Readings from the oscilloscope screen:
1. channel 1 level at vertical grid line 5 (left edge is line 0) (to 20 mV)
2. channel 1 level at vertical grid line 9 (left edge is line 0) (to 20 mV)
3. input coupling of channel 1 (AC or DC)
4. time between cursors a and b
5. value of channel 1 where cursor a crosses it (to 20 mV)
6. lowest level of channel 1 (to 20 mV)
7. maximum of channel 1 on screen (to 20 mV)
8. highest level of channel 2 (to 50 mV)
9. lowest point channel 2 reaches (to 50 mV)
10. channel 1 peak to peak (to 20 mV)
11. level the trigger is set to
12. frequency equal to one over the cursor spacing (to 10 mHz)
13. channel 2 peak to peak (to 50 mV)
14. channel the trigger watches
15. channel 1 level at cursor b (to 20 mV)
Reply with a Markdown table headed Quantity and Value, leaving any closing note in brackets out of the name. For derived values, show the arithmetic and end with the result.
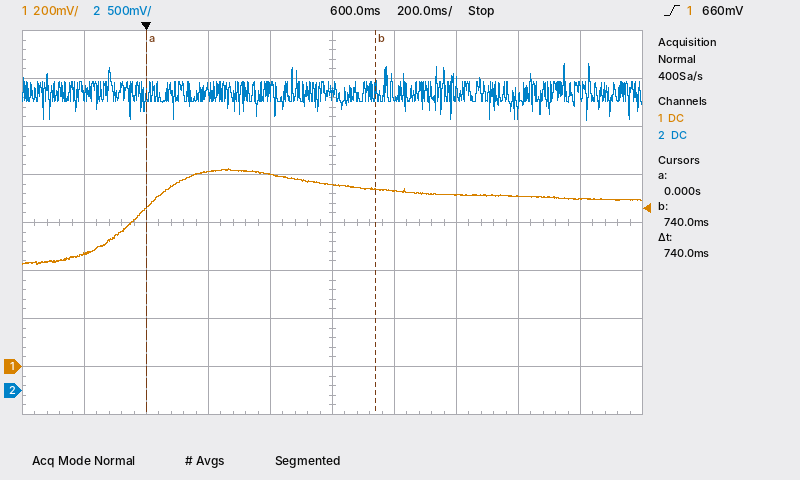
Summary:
| Quantity | Value |
|---|---|
| channel 1 level at vertical grid line 5 (left edge is line 0) | 760 mV |
| channel 1 level at vertical grid line 9 (left edge is line 0) | 700 mV |
| input coupling of channel 1 | DC |
| time between cursors a and b | 740 ms |
| value of channel 1 where cursor a crosses it | 660 mV |
| lowest level of channel 1 | 420 mV |
| maximum of channel 1 on screen | 820 mV |
| highest level of channel 2 | 3.40 V |
| lowest point channel 2 reaches | 2.80 V |
| channel 1 peak to peak | 820 mV − (420 mV) = 400 mV |
| level the trigger is set to | 660 mV |
| frequency equal to one over the cursor spacing | 1 / 740 ms ≈ 1.35 Hz |
| channel 2 peak to peak | 3.40 V − (2.80 V) = 600 mV |
| channel the trigger watches | channel 1 |
| channel 1 level at cursor b | 740 mV |
